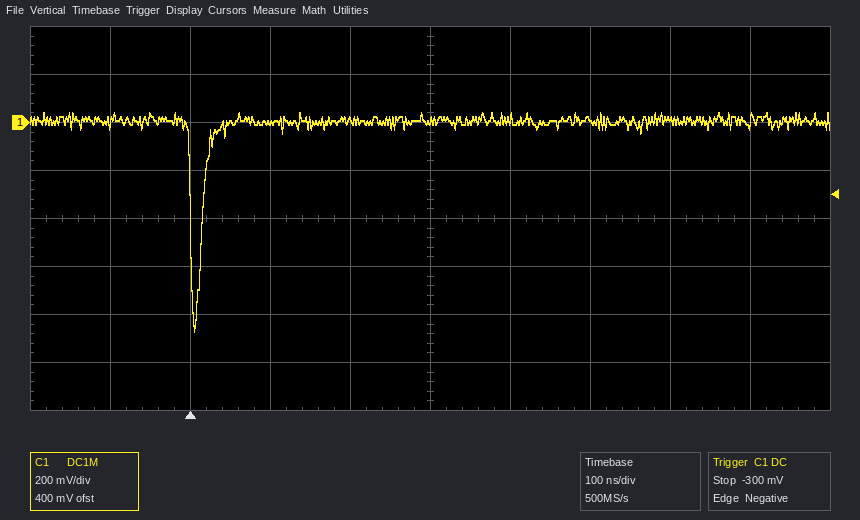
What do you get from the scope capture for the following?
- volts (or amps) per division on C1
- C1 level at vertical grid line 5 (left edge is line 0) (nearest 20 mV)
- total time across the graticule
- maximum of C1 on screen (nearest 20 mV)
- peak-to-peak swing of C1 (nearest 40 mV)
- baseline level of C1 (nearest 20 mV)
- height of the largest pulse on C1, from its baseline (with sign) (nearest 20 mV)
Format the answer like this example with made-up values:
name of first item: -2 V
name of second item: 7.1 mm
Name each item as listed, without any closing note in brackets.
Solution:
volts (or amps) per division on C1: 200 mV
C1 level at vertical grid line 5 (left edge is line 0): 0 mV
total time across the graticule: 1 µs
maximum of C1 on screen: 40 mV
peak-to-peak swing of C1: 920 mV
baseline level of C1: 0 mV
height of the largest pulse on C1, from its baseline (with sign): -880 mV
